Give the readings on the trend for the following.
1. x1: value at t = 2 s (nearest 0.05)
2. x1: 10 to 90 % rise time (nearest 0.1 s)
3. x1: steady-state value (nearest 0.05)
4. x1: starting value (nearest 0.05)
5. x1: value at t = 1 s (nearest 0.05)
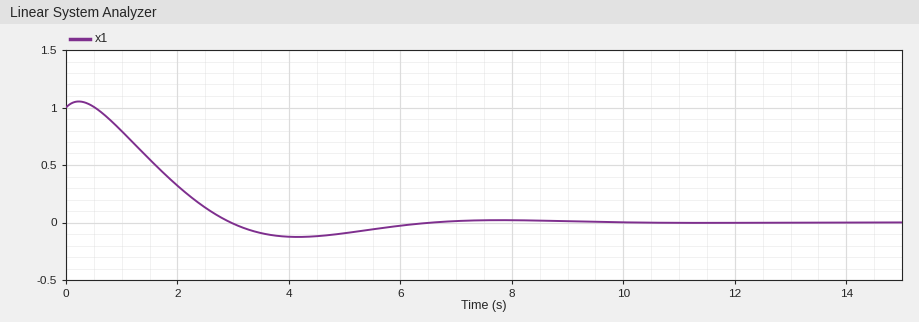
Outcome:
0.30
1.8 s
0.00
1.00
0.80
